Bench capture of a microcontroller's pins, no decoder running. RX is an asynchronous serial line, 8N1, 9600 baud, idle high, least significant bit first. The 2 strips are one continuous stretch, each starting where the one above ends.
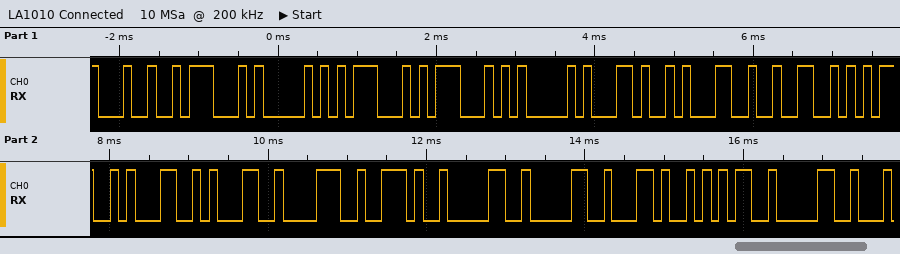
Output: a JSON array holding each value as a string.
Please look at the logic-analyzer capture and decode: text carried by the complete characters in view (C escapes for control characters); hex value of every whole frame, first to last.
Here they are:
["\"$GPGGA,125118.00,50\"", "0x24 0x47 0x50 0x47 0x47 0x41 0x2C 0x31 0x32 0x35 0x31 0x31 0x38 0x2E 0x30 0x30 0x2C 0x35 0x30"]
